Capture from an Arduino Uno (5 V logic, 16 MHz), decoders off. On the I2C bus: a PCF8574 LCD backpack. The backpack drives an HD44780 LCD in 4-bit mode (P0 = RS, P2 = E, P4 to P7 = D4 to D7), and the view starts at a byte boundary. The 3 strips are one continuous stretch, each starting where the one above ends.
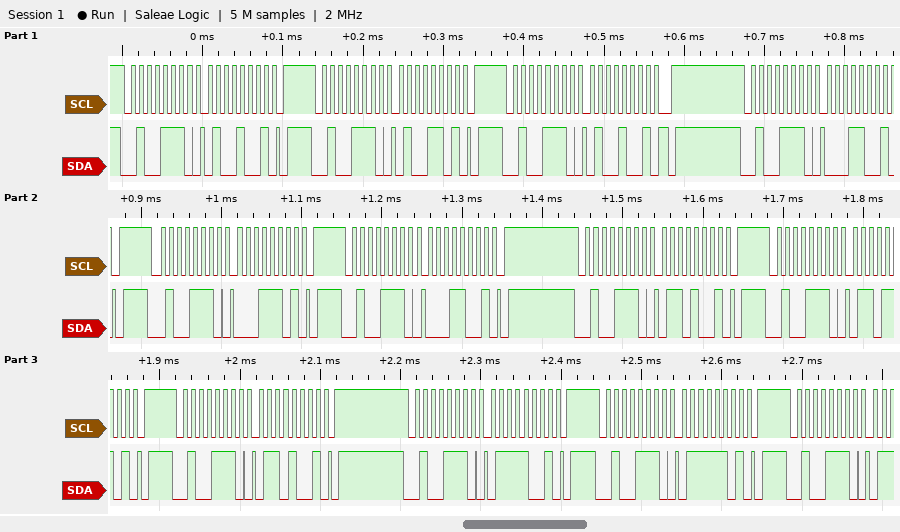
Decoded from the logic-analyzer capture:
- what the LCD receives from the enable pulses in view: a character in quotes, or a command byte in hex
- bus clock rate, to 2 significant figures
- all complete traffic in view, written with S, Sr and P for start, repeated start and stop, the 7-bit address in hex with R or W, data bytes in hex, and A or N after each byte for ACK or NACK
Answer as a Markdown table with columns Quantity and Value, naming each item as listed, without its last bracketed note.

| Quantity | Value |
|---|---|
| what the LCD receives from the enable pulses in view: a character in quotes, or a command byte in hex | 'A' |
| bus clock rate, to 2 significant figures | 100 kHz |
| all complete traffic in view, written with S, Sr and P for start, repeated start and stop, the 7-bit address in hex with R or W, data bytes in hex, and A or N after each byte for ACK or NACK | S 27W A 49 A P S 27W A 4D A P S 27W A 49 A P S 27W A 19 A P S 27W A 1D A P S 27W A 19 A P S 27W A 69 A P S 27W A 6D A P S 27W A 69 A P S 27W A 79 A P S 27W A 7D A P S 27W A |
